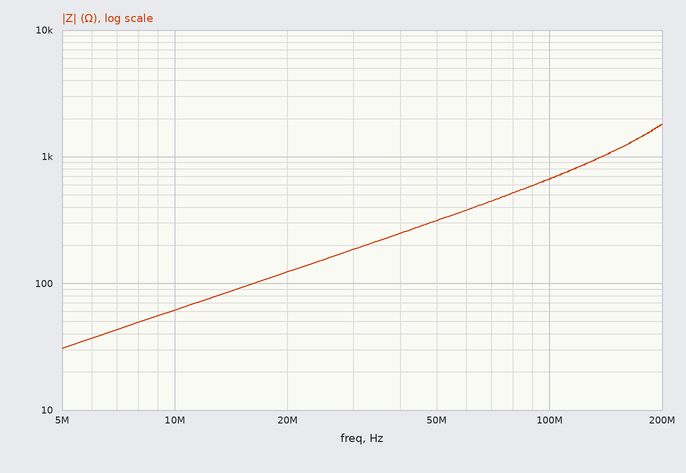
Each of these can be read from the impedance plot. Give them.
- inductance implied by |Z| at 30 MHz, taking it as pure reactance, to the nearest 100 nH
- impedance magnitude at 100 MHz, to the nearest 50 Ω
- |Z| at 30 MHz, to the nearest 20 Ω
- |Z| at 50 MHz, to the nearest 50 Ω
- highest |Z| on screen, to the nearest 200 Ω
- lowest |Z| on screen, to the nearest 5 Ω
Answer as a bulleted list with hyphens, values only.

- 1.0 µH
- 650 Ω
- 180 Ω
- 300 Ω
- 1.8 kΩ
- 30 Ω
